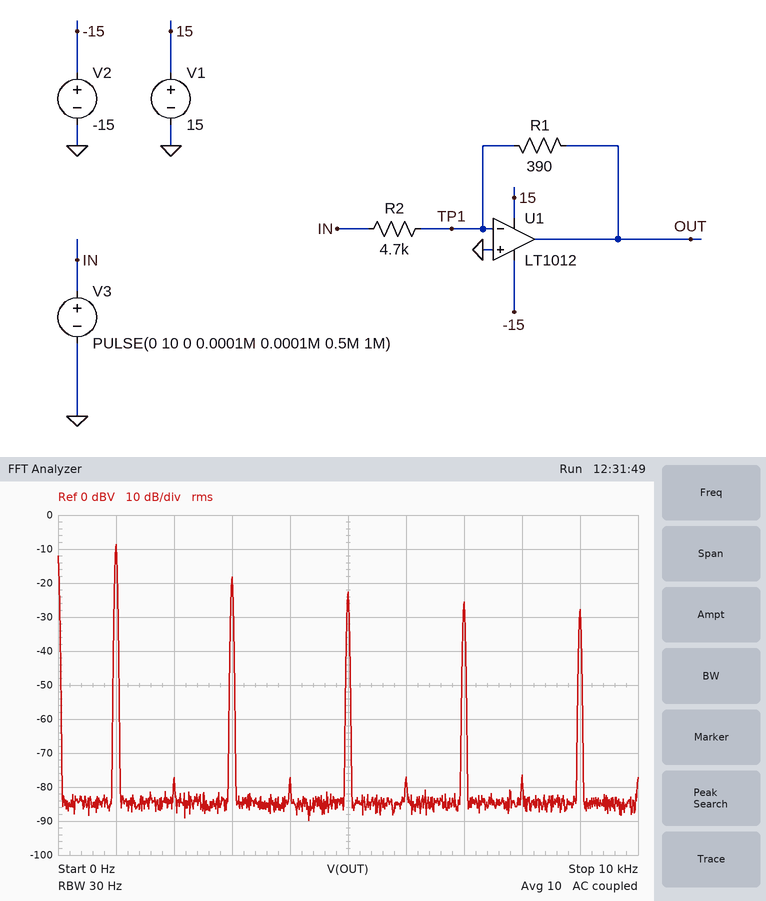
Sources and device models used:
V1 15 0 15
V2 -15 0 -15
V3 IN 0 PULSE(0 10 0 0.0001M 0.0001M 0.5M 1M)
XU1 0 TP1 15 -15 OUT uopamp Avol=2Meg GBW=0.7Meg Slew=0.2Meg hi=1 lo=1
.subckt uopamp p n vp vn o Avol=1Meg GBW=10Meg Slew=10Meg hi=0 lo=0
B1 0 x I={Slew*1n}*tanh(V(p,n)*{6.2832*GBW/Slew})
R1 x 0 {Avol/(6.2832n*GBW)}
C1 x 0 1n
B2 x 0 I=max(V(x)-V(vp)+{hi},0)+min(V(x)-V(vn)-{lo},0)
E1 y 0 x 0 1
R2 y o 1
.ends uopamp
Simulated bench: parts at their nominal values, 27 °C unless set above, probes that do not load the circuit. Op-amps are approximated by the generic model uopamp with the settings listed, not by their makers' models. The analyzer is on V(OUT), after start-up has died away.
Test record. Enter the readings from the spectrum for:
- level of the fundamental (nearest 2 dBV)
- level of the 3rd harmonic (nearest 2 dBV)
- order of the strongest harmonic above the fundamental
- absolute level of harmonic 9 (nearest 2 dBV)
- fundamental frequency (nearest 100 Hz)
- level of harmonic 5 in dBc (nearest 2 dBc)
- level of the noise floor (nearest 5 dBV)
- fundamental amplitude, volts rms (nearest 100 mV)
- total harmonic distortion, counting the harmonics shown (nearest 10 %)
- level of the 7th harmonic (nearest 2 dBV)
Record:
-8 dBV
-18 dBV
3
-28 dBV
1.0 kHz
-14 dBc
-85 dBV
400 mV
40 %
-26 dBV
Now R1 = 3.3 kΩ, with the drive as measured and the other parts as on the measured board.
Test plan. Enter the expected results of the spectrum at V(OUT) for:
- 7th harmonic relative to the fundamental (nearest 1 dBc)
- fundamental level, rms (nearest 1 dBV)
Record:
-18 dBc
10 dBV
